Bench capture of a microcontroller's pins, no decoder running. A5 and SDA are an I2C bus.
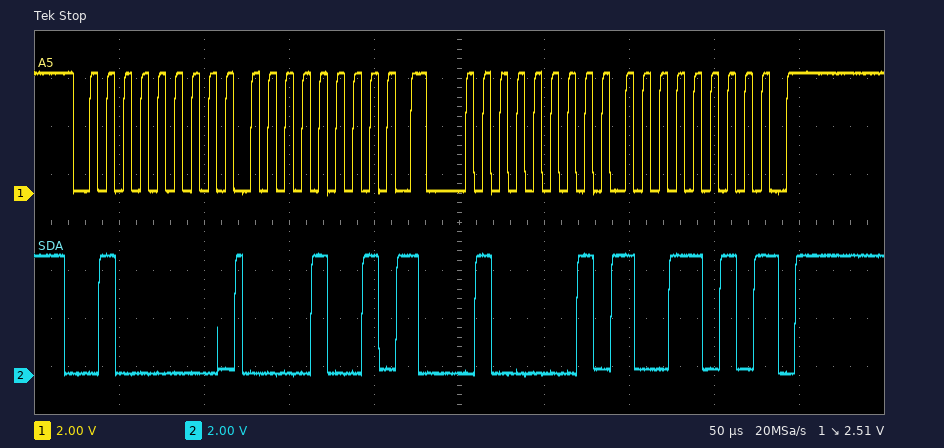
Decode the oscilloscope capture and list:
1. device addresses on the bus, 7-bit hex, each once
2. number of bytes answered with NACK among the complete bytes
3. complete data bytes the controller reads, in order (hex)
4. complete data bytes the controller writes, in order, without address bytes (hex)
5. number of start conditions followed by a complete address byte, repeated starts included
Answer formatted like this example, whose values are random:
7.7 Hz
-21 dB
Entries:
0x20
1
9A
09
2
